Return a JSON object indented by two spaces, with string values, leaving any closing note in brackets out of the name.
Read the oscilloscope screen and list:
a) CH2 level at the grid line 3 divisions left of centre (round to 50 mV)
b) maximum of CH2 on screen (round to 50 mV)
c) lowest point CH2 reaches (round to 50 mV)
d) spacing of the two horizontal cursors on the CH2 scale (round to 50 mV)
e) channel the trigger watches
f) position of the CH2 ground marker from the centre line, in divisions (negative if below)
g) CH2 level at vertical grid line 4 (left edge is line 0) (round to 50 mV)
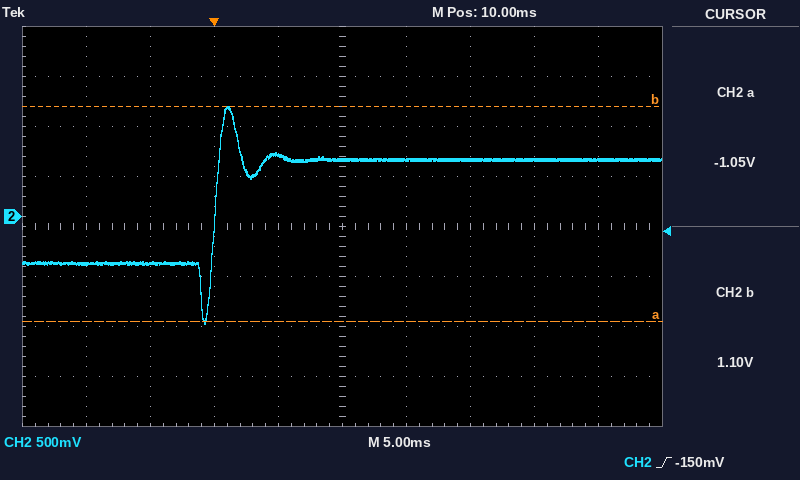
{
  "CH2 level at the grid line 3 divisions left of centre": "-450 mV",
  "maximum of CH2 on screen": "1.10 V",
  "lowest point CH2 reaches": "-1.05 V",
  "spacing of the two horizontal cursors on the CH2 scale": "2.15 V",
  "channel the trigger watches": "CH2",
  "position of the CH2 ground marker from the centre line, in divisions": "+0.2 div",
  "CH2 level at vertical grid line 4 (left edge is line 0)": "600 mV"
}
